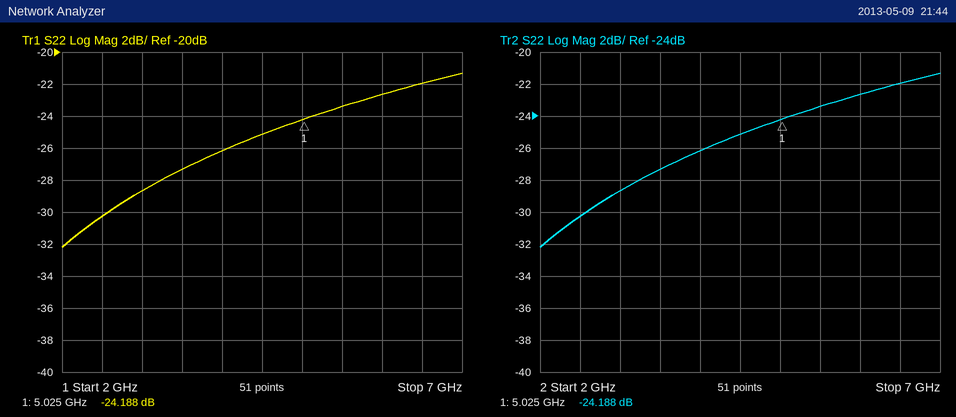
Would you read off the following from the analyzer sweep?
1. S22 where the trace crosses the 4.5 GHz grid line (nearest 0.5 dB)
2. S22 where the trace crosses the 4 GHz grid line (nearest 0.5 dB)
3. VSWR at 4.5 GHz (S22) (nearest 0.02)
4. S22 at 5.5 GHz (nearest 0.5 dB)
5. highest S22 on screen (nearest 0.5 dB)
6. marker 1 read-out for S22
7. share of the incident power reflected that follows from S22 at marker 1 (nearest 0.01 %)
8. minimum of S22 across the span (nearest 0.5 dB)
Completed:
-25.0 dB
-26.0 dB
1.12
-23.5 dB
-21.5 dB
-24.188 dB
0.38 %
-32.0 dB
